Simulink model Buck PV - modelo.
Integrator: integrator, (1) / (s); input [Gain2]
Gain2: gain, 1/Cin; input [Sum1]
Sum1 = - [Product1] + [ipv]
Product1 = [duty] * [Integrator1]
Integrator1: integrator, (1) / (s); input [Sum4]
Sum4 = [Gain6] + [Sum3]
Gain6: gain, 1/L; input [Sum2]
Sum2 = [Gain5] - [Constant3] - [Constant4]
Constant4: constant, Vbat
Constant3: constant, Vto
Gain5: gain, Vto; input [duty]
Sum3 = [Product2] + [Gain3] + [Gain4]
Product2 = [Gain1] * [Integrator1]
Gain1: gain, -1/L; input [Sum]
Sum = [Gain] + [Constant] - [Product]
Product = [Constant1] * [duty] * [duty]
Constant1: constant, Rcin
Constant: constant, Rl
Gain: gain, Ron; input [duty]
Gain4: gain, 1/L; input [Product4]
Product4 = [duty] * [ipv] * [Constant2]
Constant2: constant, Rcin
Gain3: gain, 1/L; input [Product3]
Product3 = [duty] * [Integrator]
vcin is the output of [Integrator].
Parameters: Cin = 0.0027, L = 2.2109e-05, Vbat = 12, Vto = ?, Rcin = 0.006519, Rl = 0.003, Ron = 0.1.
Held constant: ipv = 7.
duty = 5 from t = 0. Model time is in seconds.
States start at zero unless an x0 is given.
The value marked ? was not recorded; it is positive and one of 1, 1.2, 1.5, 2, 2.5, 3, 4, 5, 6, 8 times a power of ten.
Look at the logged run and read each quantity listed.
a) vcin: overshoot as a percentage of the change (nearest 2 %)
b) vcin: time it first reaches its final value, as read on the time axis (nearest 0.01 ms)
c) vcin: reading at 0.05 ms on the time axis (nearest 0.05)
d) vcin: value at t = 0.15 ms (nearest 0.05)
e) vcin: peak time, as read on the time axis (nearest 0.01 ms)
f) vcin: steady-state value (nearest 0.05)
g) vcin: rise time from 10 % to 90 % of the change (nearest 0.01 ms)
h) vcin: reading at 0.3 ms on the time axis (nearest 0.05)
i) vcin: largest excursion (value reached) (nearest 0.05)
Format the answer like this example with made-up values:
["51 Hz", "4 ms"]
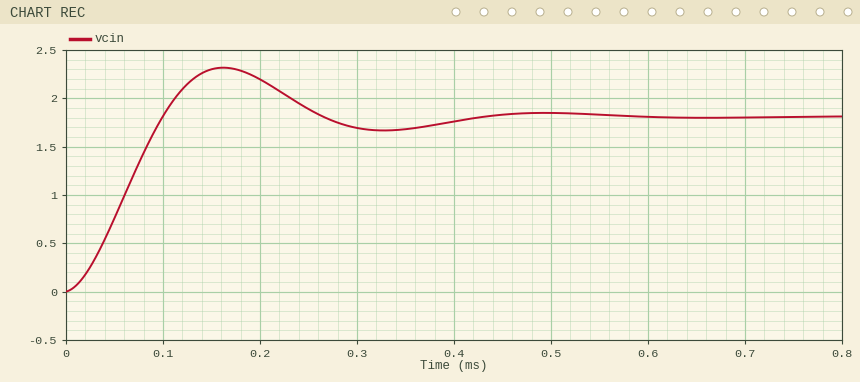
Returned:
["28 %", "0.10 ms", "0.75", "2.30", "0.16 ms", "1.80", "0.07 ms", "1.70", "2.30"]
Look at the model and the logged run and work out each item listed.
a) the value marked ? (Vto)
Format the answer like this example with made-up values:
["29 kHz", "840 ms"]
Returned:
["0.8"]
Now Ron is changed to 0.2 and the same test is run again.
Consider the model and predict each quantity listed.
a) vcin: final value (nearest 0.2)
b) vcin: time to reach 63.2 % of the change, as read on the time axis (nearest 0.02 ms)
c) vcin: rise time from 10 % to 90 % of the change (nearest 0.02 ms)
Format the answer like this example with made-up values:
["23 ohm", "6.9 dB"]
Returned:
["2.0", "0.10 ms", "0.14 ms"]
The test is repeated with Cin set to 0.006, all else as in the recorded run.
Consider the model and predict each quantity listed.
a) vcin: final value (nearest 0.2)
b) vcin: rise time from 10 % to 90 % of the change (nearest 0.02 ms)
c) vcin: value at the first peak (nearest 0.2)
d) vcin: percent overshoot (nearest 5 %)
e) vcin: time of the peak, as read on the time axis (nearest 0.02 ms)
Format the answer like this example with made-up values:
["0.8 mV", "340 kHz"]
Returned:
["1.8", "0.12 ms", "2.0", "10 %", "0.28 ms"]
